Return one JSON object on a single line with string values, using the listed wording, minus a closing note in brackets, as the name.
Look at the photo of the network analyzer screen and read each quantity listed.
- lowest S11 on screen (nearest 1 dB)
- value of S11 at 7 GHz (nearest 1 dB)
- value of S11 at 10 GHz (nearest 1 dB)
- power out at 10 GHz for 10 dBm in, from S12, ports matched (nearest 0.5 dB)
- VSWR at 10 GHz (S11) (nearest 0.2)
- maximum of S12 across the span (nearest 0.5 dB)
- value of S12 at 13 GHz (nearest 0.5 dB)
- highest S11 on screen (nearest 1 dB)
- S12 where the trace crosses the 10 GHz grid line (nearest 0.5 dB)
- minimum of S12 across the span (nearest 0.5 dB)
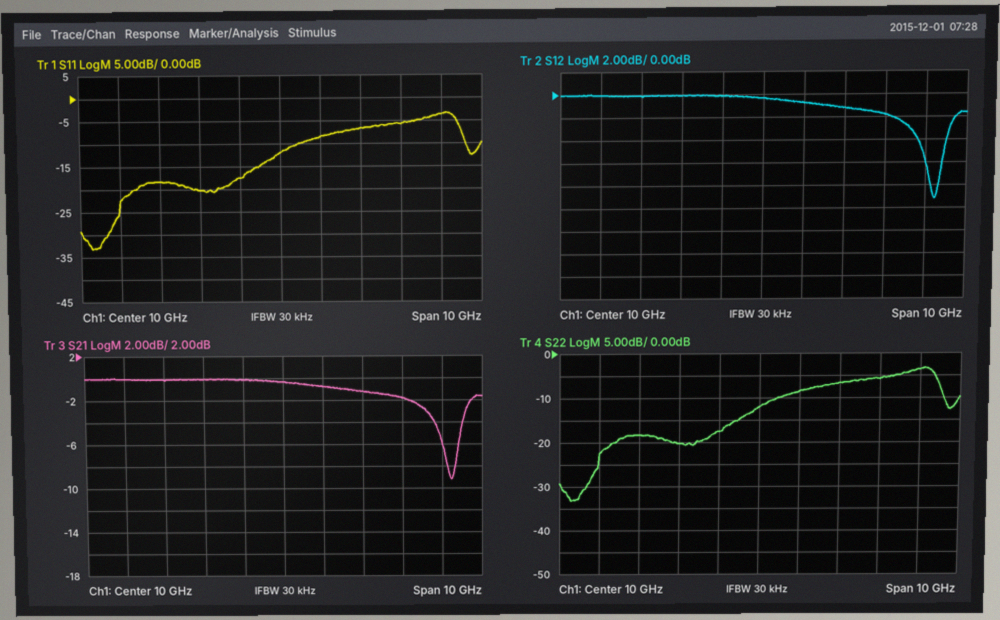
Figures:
{"lowest S11 on screen": "-33 dB", "value of S11 at 7 GHz": "-18 dB", "value of S11 at 10 GHz": "-12 dB", "power out at 10 GHz for 10 dBm in, from S12, ports matched": "9.5 dBm", "VSWR at 10 GHz (S11)": "1.6", "maximum of S12 across the span": "0.0 dB", "value of S12 at 13 GHz": "-2.0 dB", "highest S11 on screen": "-3 dB", "S12 where the trace crosses the 10 GHz grid line": "-0.5 dB", "minimum of S12 across the span": "-9.0 dB"}
